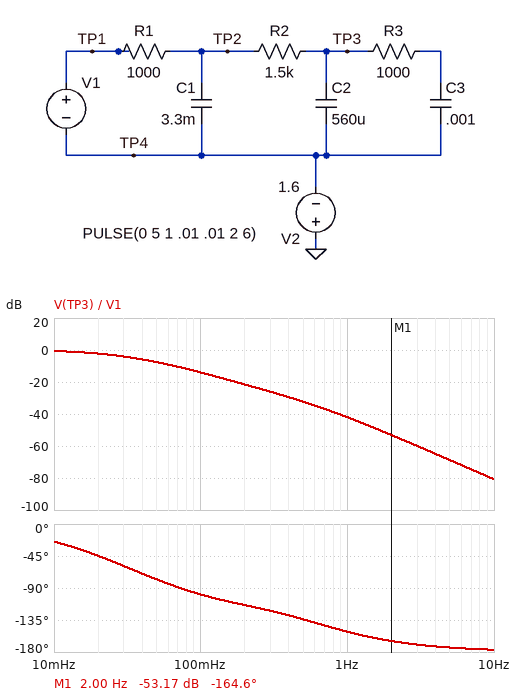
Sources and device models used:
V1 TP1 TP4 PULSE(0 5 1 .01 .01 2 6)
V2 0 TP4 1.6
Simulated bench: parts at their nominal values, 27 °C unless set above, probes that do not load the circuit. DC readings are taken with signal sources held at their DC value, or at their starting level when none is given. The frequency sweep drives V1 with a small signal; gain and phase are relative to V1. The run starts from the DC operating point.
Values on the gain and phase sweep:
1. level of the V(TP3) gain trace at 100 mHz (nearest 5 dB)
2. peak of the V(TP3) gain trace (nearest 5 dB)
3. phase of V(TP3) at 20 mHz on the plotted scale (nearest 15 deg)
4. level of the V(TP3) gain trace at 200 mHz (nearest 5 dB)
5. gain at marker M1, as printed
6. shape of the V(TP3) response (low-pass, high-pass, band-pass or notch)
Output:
-15 dB
0 dB
-45 deg
-20 dB
-53.17 dB
low-pass
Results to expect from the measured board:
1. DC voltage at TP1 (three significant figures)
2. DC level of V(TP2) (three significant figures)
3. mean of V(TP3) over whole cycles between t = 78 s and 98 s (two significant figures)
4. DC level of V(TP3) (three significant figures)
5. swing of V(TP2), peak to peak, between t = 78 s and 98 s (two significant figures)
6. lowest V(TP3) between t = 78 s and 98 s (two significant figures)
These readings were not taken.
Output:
-1.60 V
-1.60 V
75 mV
-1.60 V
1.7 V
-260 mV
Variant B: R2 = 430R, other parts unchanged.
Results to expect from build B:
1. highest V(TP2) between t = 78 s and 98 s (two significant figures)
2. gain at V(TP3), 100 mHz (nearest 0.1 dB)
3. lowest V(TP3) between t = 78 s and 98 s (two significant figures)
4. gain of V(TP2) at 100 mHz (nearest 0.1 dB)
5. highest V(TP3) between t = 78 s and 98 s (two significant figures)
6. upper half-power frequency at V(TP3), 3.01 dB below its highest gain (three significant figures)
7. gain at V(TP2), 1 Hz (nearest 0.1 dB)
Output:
960 mV
-11.0 dB
-470 mV
-9.6 dB
670 mV
29.5 mHz
-26.7 dB
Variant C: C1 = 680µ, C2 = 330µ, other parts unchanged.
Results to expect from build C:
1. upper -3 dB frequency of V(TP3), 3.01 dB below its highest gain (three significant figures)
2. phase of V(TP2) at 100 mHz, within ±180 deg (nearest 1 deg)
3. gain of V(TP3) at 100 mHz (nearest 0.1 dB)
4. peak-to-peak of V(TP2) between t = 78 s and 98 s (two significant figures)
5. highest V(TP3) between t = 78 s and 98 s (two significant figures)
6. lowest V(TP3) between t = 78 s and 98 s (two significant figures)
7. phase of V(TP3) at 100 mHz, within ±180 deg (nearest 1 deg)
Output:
37.9 mHz
-26 deg
-8.3 dB
3.6 V
1.1 V
-710 mV
-60 deg
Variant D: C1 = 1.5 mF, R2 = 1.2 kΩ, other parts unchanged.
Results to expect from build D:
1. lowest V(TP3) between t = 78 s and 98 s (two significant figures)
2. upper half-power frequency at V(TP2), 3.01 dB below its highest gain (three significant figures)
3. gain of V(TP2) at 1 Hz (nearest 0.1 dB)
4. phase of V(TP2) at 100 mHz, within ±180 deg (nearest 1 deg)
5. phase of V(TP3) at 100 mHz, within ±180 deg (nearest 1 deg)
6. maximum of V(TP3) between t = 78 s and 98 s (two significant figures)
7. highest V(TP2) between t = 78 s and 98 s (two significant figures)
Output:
-540 mV
46.3 mHz
-19.8 dB
-41 deg
-77 deg
770 mV
1.7 V
